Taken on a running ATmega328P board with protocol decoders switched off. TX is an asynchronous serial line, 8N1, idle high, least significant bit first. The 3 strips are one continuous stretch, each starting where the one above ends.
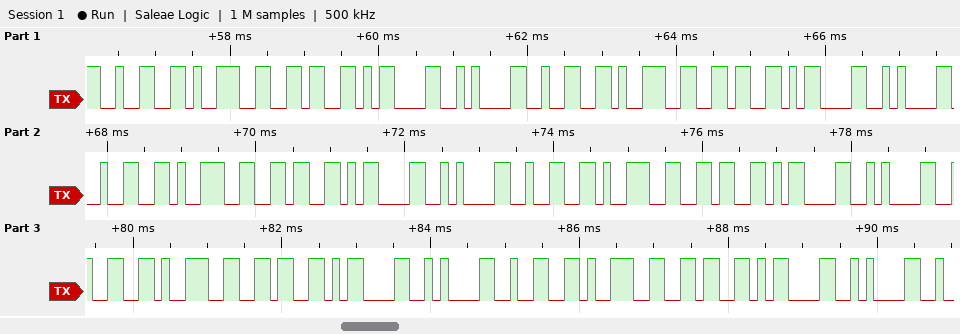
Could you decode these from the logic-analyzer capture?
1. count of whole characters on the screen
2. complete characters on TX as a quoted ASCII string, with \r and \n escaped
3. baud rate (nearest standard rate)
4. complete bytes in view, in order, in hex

30
"296\r\n296\r\n296\r\n296\r\n296\r\n296\r\n"
9600 baud
32 39 36 0D 0A 32 39 36 0D 0A 32 39 36 0D 0A 32 39 36 0D 0A 32 39 36 0D 0A 32 39 36 0D 0A
